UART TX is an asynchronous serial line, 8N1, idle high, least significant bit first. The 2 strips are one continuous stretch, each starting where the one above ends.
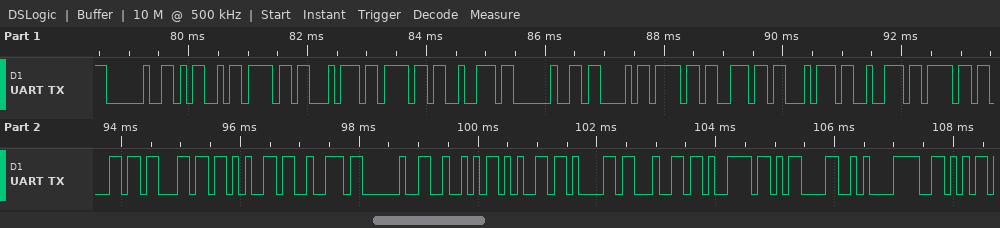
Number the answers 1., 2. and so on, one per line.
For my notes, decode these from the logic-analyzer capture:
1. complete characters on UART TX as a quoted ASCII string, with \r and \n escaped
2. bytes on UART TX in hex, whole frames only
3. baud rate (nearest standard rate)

1. " Motor Controller Ready\r\nV"
2. 20 4D 6F 74 6F 72 20 43 6F 6E 74 72 6F 6C 6C 65 72 20 52 65 61 64 79 0D 0A 56
3. 9600 baud
